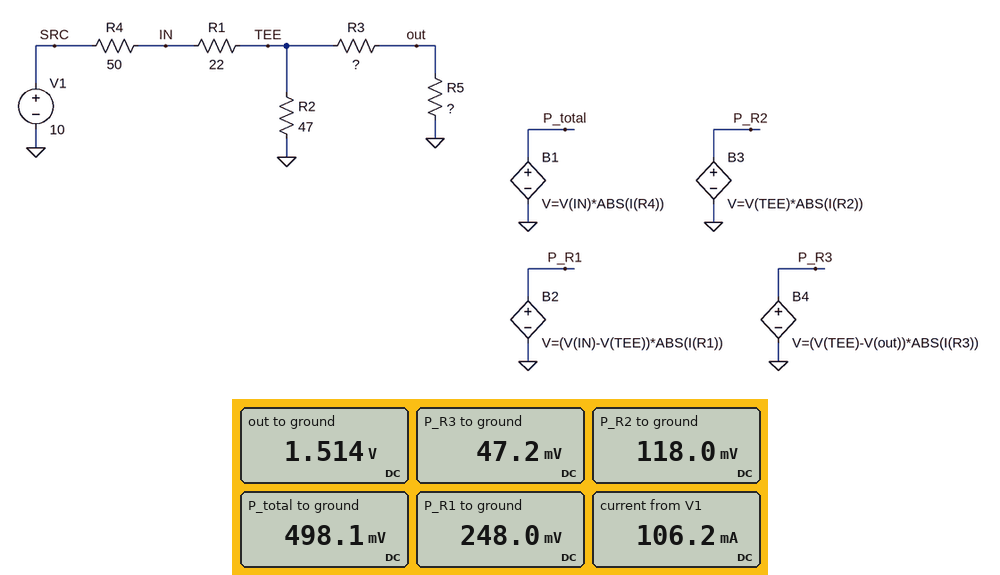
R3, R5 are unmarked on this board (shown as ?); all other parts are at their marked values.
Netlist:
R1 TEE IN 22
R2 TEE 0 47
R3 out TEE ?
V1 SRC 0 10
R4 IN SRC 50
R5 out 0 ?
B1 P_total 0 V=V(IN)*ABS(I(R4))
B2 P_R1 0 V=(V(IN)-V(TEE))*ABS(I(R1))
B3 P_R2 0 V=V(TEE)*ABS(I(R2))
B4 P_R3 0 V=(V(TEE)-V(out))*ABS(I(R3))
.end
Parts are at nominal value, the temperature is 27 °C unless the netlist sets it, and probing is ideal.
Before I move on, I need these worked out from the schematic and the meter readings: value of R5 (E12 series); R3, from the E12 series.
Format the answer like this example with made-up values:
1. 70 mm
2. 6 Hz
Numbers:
1. 27 Ω
2. 15 Ω
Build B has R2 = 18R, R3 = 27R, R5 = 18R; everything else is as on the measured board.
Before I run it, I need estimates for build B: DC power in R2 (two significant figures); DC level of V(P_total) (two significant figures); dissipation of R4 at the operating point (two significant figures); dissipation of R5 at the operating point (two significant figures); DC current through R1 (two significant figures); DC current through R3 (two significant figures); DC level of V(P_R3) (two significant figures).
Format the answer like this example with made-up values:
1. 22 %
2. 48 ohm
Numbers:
1. 130 mW
2. 480 mV
3. 690 mW
4. 20 mW
5. 120 mA
6. 34 mA
7. 31 mV
